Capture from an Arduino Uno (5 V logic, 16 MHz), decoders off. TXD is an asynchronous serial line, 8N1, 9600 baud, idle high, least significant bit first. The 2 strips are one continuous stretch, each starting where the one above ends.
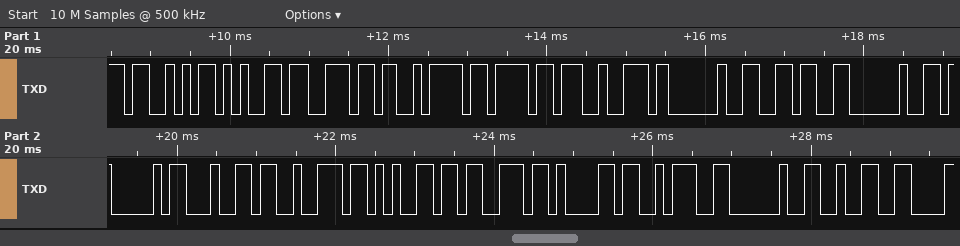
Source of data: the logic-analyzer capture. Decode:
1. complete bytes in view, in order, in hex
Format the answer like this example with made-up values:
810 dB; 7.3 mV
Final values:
53 65 6E 7A 6F 72 20 36 20 41 64 72 65 73 61 3A 20 32
